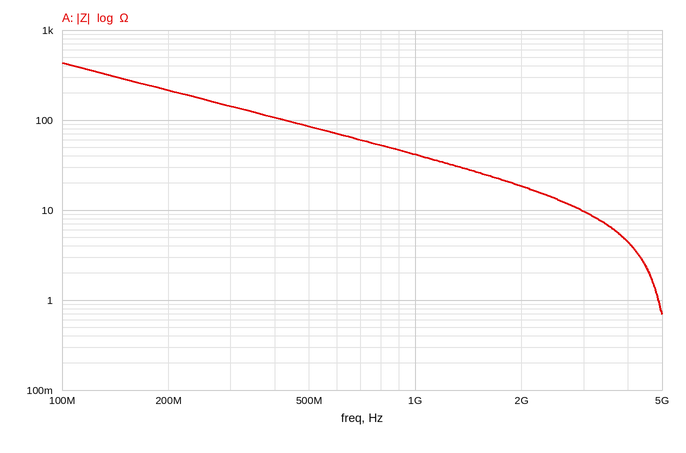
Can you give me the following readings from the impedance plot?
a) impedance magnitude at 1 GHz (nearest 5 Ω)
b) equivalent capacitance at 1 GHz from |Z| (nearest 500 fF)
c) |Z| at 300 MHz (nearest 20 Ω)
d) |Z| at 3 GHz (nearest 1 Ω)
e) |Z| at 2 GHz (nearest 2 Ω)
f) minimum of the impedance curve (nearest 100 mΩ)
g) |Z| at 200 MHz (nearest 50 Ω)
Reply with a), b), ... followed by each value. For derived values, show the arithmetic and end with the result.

a) 40 Ω
b) C = 1/(2π × 1 GHz × 40 Ω) ≈ 4.0 pF
c) 140 Ω
d) 10 Ω
e) 18 Ω
f) 700 mΩ
g) 200 Ω
